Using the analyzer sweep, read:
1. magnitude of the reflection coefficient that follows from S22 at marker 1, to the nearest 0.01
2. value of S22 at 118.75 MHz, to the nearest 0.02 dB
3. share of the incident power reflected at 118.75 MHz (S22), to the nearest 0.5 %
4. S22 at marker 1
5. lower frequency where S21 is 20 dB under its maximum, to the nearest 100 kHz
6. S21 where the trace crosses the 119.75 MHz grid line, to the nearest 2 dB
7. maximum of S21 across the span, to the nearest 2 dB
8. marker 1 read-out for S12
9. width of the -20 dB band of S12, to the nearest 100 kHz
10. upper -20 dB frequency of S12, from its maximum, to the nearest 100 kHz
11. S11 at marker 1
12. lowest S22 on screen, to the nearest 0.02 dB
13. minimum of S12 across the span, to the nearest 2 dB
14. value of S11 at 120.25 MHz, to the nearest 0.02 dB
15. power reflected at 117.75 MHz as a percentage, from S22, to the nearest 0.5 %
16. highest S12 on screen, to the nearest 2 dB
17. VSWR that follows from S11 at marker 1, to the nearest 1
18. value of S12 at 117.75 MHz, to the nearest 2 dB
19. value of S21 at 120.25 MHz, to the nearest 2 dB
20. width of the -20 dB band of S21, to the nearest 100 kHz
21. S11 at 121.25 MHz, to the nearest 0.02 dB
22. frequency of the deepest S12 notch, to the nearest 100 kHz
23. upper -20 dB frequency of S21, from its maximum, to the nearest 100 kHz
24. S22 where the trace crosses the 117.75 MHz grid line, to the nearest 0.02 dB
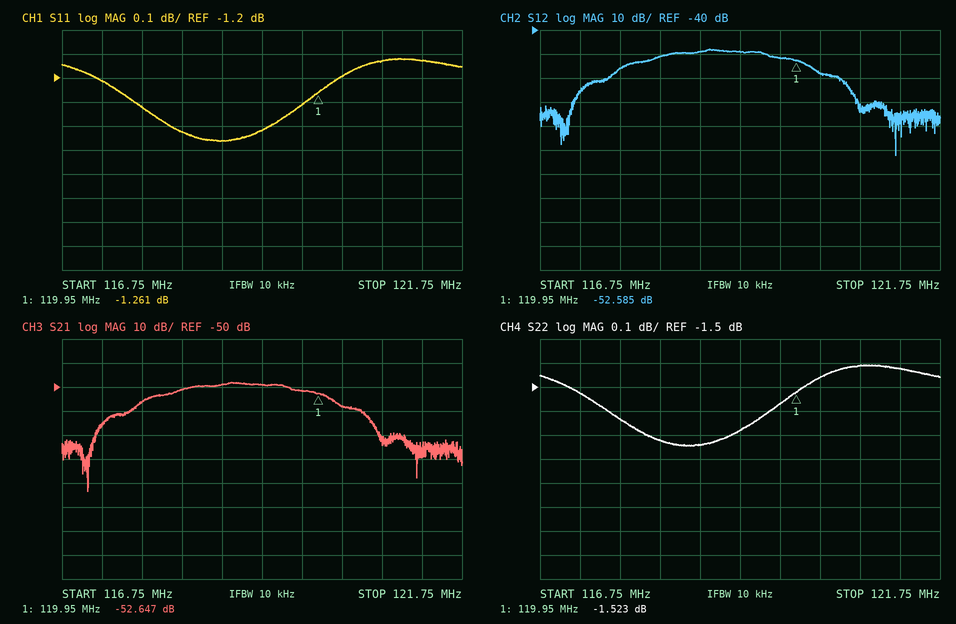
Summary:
0.84
-1.74 dB
67.0 %
-1.523 dB
117.2 MHz
-52 dB
-48 dB
-52.585 dB
3.5 MHz
120.7 MHz
-1.261 dB
-1.74 dB
-92 dB
-1.20 dB
68.5 %
-48 dB
14
-56 dB
-58 dB
3.5 MHz
-1.12 dB
121.2 MHz
120.7 MHz
-1.64 dB
